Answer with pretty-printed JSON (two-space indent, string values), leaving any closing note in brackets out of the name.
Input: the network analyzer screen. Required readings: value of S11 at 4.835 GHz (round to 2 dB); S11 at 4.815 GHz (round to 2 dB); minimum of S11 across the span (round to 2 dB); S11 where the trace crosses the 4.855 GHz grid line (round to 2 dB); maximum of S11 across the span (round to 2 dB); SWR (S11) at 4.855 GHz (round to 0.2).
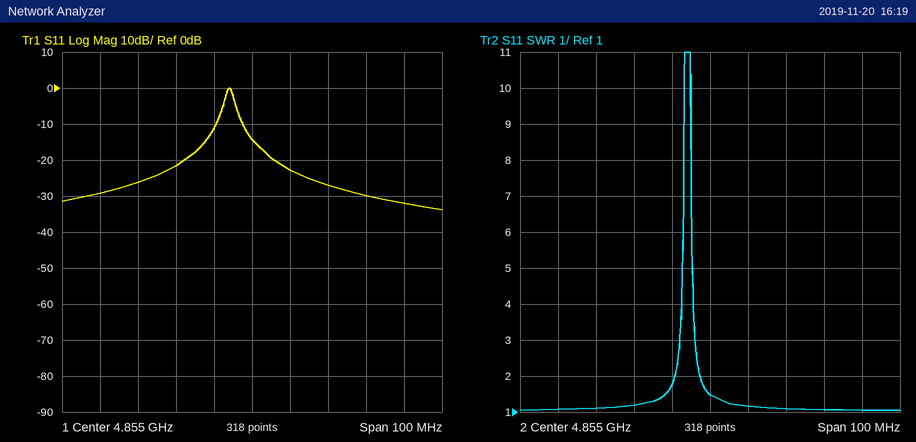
{
  "value of S11 at 4.835 GHz": "-22 dB",
  "S11 at 4.815 GHz": "-30 dB",
  "minimum of S11 across the span": "-34 dB",
  "S11 where the trace crosses the 4.855 GHz grid line": "-14 dB",
  "maximum of S11 across the span": "0 dB",
  "SWR (S11) at 4.855 GHz": "1.4"
}
